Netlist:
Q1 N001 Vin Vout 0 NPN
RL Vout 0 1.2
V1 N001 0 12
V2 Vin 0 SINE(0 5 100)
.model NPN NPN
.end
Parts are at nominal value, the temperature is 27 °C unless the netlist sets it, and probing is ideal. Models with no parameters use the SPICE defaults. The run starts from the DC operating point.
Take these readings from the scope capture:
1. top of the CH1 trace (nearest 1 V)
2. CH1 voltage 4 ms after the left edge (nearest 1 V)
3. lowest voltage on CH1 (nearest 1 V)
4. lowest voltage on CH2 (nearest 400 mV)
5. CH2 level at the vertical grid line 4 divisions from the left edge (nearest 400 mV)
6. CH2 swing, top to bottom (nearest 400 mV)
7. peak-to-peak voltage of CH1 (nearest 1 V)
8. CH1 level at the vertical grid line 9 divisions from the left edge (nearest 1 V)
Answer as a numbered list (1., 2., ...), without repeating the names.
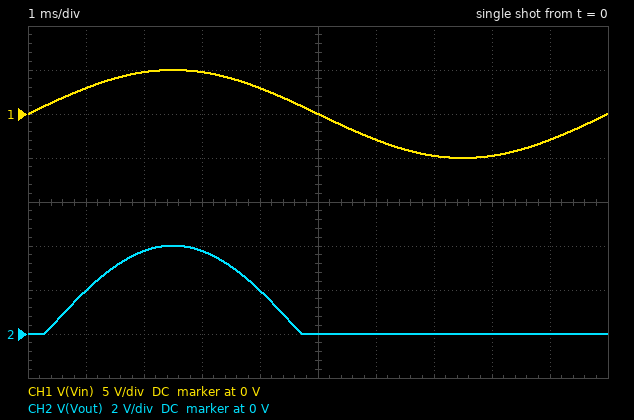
1. 5 V
2. 3 V
3. -5 V
4. 0 V
5. 2.0 V
6. 4.0 V
7. 10 V
8. -3 V
